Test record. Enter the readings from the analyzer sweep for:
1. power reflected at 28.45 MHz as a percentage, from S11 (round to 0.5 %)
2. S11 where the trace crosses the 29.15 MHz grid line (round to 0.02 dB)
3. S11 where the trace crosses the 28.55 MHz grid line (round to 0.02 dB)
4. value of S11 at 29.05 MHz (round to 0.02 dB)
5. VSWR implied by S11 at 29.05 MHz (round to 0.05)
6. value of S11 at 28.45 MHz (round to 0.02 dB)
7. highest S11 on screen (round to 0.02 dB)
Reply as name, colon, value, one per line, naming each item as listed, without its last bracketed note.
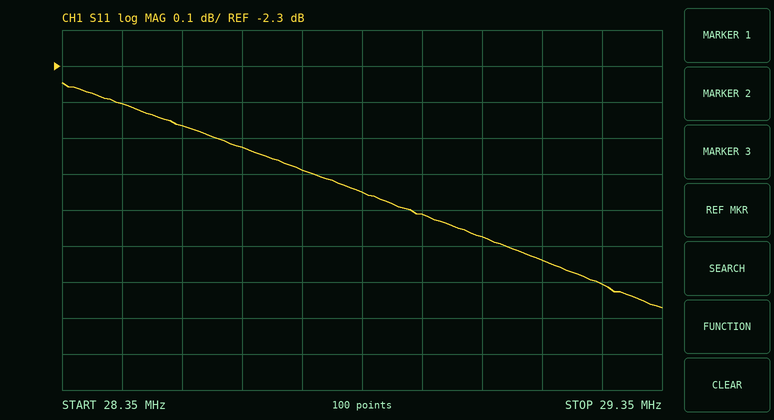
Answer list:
power reflected at 28.45 MHz as a percentage, from S11: 57.5 %
S11 where the trace crosses the 29.15 MHz grid line: -2.84 dB
S11 where the trace crosses the 28.55 MHz grid line: -2.46 dB
value of S11 at 29.05 MHz: -2.78 dB
VSWR implied by S11 at 29.05 MHz: 6.30
value of S11 at 28.45 MHz: -2.40 dB
highest S11 on screen: -2.34 dB
